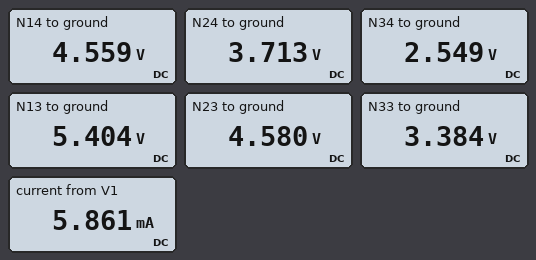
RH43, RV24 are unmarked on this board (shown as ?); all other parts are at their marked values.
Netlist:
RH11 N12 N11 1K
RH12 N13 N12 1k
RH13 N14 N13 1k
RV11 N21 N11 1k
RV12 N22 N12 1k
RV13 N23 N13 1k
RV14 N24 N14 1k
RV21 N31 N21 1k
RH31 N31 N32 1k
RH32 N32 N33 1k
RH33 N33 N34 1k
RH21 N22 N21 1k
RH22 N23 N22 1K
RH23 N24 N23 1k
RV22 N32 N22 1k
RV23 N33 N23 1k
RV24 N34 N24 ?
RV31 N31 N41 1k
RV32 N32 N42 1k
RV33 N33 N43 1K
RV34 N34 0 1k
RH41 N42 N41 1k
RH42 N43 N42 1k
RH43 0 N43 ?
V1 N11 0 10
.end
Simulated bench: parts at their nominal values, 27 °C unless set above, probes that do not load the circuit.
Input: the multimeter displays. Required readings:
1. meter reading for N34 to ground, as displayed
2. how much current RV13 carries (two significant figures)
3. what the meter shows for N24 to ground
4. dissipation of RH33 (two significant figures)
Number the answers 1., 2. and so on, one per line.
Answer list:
1. 2.549 V
2. 820 µA
3. 3.713 V
4. 700 µW
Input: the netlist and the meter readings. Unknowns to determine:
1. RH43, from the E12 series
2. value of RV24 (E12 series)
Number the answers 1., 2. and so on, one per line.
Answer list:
1. 560 Ω
2. 680 Ω
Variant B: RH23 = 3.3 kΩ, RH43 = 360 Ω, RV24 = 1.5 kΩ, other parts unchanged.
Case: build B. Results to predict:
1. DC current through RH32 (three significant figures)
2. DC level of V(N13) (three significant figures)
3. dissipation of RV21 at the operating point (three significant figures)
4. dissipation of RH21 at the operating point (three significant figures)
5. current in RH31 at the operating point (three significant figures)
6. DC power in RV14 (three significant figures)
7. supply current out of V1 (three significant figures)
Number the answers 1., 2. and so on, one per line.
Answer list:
1. 1.23 mA
2. 5.49 V
3. 3.19 mW
4. 1.46 mW
5. 845 µA
6. 706 µW
7. 5.90 mA
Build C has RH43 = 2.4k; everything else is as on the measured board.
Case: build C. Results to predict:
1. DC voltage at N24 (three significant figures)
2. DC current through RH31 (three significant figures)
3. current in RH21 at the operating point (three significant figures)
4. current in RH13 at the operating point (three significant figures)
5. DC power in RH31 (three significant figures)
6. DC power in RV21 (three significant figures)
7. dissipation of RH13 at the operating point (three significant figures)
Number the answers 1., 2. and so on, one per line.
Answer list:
1. 4.40 V
2. 692 µA
3. 1.08 mA
4. 822 µA
5. 479 µW
6. 1.68 mW
7. 675 µW
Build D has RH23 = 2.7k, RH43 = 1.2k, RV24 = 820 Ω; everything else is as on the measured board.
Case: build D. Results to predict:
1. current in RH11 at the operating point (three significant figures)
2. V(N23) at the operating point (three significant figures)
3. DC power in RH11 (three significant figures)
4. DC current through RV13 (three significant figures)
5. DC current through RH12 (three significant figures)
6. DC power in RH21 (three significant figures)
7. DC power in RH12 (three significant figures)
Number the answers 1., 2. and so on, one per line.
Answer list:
1. 2.63 mA
2. 5.22 V
3. 6.92 mW
4. 599 µA
5. 1.55 mA
6. 1.24 mW
7. 2.41 mW
